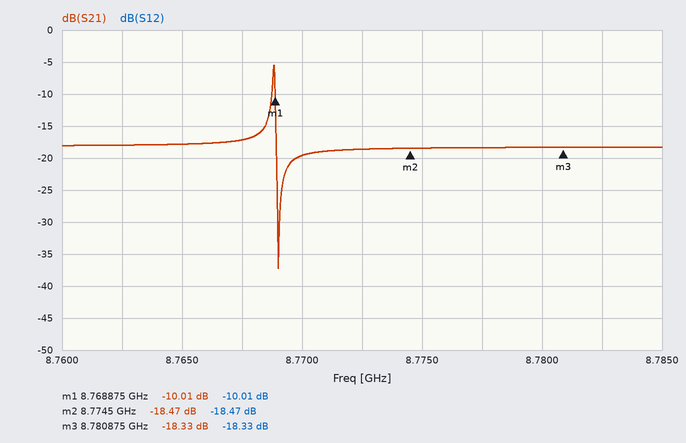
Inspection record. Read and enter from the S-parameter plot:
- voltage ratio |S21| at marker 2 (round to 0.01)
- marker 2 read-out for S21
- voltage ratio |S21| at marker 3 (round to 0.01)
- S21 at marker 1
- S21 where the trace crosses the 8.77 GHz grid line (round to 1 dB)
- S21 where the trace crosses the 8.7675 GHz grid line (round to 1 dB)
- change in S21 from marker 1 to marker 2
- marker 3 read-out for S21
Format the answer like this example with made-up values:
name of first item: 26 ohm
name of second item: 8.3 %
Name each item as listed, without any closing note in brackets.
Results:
voltage ratio |S21| at marker 2: 0.12
marker 2 read-out for S21: -18.47 dB
voltage ratio |S21| at marker 3: 0.12
S21 at marker 1: -10.01 dB
S21 where the trace crosses the 8.77 GHz grid line: -20 dB
S21 where the trace crosses the 8.7675 GHz grid line: -17 dB
change in S21 from marker 1 to marker 2: -8.46 dB
marker 3 read-out for S21: -18.33 dB
